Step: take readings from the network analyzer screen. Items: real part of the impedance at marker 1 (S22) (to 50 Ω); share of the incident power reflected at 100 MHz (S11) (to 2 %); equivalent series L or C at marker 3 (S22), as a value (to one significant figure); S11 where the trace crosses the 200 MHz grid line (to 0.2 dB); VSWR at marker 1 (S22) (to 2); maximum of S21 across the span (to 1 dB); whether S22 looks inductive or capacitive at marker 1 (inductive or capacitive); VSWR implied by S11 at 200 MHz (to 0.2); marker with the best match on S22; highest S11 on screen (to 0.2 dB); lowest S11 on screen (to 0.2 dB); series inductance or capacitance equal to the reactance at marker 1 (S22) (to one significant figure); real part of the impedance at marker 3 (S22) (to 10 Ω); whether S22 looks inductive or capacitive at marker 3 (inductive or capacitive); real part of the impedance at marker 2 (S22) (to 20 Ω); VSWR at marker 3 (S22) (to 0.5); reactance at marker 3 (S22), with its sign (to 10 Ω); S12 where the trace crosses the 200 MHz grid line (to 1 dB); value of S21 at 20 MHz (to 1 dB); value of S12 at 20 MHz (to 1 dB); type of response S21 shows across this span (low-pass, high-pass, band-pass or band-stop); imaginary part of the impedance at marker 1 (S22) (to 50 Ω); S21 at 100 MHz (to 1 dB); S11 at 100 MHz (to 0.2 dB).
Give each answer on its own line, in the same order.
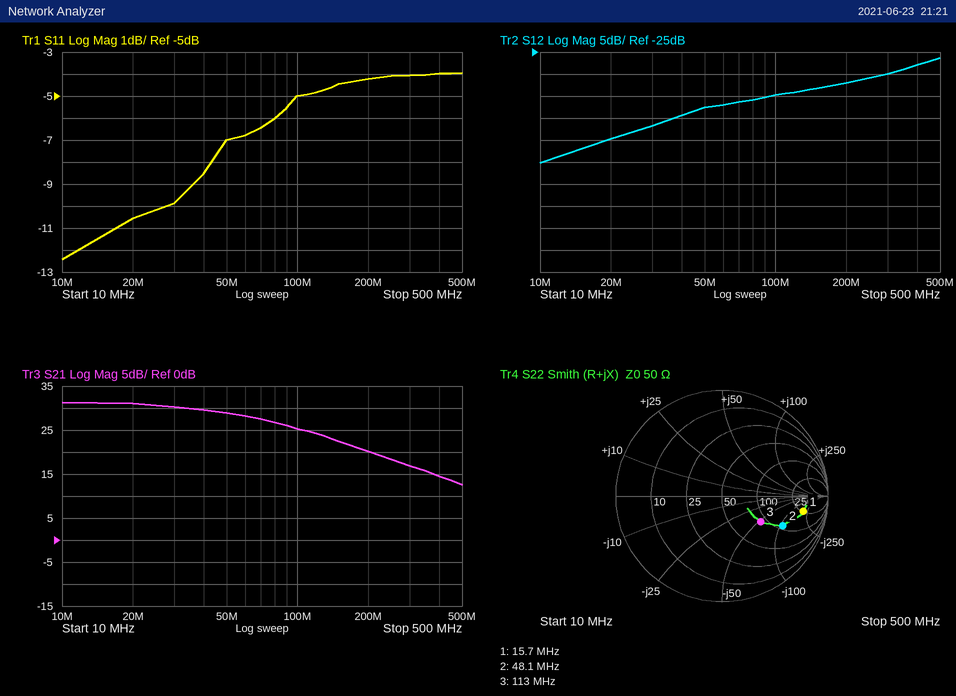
250 Ω
32 %
30 pF
-4.2 dB
8
31 dB
capacitive
4.2
marker 3
-4.0 dB
-12.4 dB
50 pF
90 Ω
capacitive
120 Ω
2.5
-50 Ω
-32 dB
31 dB
-45 dB
low-pass
-200 Ω
25 dB
-5.0 dB
